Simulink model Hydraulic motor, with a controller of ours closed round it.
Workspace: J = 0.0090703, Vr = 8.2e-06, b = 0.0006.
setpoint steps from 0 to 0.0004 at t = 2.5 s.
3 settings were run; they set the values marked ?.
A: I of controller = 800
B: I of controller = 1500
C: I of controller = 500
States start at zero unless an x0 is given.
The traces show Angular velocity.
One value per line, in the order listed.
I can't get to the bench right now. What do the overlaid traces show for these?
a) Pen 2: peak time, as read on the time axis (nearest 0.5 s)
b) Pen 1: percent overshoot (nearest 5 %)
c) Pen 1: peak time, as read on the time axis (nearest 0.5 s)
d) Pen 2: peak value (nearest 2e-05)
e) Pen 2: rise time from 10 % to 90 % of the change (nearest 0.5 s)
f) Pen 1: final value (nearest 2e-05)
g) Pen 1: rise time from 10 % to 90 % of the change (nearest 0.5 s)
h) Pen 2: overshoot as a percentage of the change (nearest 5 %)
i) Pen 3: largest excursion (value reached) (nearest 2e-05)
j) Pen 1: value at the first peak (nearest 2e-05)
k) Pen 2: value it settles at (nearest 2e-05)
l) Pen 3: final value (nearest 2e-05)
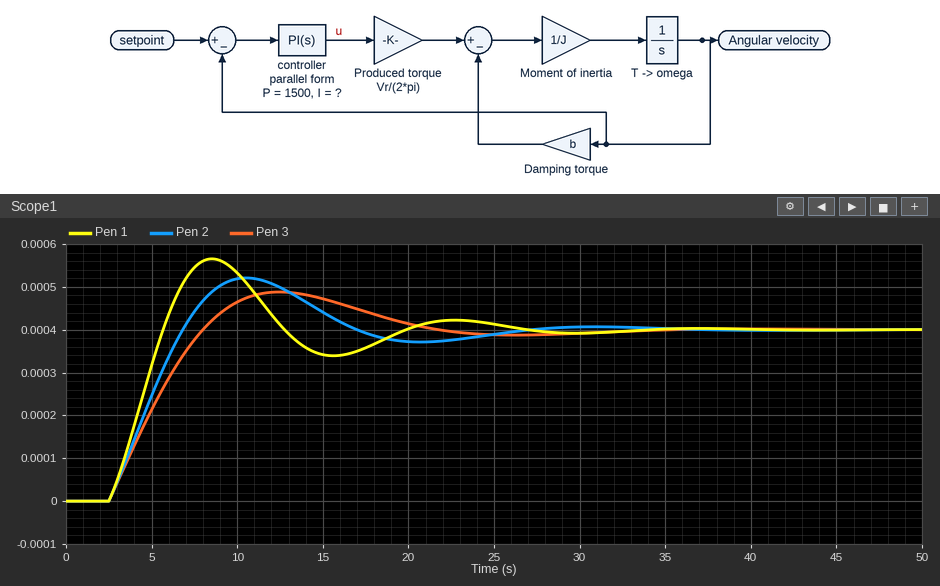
10.5 s
40 %
8.5 s
0.00052
3.5 s
0.00040
2.5 s
30 %
0.00048
0.00056
0.00040
0.00040
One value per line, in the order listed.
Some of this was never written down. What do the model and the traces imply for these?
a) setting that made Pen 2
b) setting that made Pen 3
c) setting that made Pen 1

A
C
B
